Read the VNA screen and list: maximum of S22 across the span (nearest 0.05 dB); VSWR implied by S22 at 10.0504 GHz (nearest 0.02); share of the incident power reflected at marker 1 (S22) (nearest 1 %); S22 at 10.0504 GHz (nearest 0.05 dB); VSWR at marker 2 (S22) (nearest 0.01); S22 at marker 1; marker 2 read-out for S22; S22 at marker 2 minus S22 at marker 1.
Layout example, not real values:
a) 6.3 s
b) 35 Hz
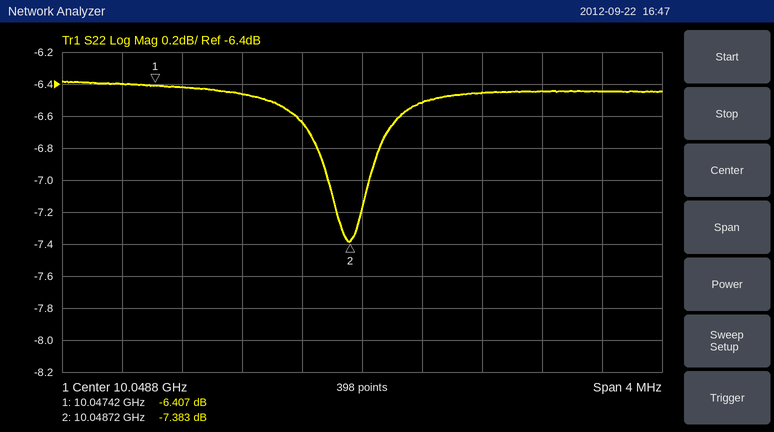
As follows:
a) -6.40 dB
b) 2.82
c) 23 %
d) -6.45 dB
e) 2.49
f) -6.407 dB
g) -7.383 dB
h) -0.976 dB
